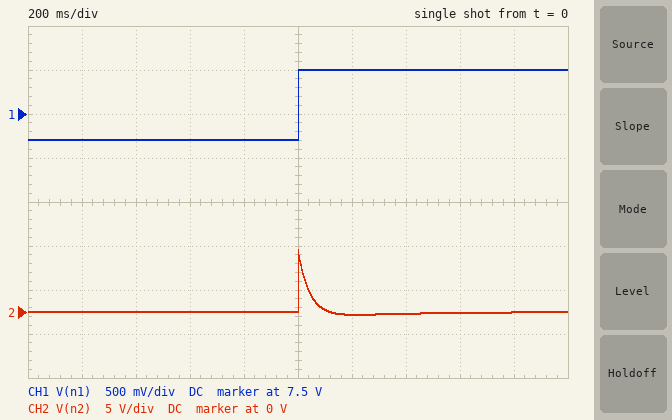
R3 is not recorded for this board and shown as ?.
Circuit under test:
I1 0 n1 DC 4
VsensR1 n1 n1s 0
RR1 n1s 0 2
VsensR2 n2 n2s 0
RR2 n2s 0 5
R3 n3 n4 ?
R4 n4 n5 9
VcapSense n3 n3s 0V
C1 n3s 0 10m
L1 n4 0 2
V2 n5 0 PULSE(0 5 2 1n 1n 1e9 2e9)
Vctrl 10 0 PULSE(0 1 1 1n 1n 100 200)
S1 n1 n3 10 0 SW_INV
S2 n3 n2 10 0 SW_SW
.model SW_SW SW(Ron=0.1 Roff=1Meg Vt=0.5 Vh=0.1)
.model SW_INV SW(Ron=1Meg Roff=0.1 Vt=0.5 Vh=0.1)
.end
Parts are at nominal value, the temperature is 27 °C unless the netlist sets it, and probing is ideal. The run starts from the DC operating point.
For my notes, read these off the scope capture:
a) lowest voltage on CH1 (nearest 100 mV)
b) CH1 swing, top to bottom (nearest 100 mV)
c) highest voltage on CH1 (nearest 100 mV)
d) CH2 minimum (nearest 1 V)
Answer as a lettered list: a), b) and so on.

a) 7.2 V
b) 800 mV
c) 8.0 V
d) 0 V
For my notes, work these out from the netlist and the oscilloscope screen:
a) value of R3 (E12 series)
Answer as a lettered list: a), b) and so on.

a) 18 Ω
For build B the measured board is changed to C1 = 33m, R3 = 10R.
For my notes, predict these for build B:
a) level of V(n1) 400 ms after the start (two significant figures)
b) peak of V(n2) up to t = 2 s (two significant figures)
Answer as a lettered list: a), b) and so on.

a) 6.7 V
b) 6.5 V
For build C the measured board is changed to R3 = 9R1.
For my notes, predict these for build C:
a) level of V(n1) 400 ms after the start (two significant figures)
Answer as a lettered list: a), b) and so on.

a) 6.6 V
